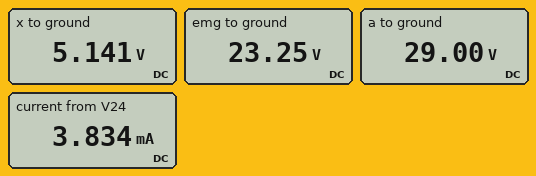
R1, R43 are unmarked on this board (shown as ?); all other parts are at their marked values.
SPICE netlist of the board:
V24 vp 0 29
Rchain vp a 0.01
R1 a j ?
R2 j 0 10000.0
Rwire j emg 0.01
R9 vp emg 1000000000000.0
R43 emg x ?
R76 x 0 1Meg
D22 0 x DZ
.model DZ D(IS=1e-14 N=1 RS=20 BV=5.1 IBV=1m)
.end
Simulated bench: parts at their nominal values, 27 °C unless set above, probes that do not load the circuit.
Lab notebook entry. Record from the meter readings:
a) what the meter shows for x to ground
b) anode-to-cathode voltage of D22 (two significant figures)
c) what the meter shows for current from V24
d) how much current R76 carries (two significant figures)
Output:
5.141 V
-5.1 V
3.834 mA
5.1 µA
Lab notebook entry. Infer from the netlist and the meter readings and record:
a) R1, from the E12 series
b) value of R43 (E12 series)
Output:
1.5 kΩ
12 kΩ
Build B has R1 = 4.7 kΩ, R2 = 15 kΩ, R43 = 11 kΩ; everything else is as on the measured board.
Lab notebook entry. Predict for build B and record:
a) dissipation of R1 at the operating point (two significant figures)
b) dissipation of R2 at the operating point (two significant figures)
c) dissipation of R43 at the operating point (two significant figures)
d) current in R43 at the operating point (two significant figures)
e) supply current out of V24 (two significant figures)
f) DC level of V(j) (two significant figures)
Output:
26 mW
21 mW
15 mW
1.2 mA
2.4 mA
18 V
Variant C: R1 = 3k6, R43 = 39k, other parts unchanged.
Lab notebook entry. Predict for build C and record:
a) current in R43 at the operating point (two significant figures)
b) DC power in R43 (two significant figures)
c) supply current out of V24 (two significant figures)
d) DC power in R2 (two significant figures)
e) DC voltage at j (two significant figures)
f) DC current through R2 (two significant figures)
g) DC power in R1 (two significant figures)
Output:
390 µA
5.9 mW
2.4 mA
41 mW
20 V
2.0 mA
21 mW
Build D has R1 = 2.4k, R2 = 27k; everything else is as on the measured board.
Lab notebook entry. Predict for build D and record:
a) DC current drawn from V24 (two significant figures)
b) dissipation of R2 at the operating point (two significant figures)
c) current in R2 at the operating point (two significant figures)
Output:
2.4 mA
20 mW
860 µA
